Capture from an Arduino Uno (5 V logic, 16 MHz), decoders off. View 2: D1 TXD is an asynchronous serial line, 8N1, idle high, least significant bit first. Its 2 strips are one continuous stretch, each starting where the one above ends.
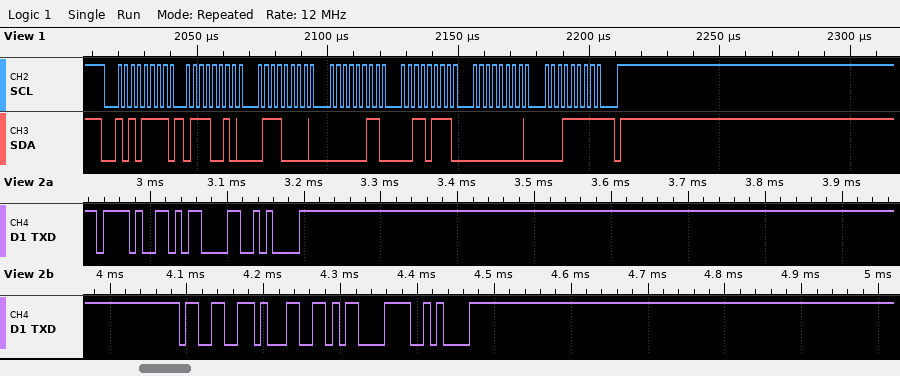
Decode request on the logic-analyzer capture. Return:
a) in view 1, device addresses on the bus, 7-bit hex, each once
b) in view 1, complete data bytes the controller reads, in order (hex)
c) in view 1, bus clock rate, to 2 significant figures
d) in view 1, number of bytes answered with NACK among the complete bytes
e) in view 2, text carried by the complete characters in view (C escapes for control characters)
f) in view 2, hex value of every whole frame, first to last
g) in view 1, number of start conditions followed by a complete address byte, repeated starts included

0x57
72 70 03 37 00 1F
400 kHz
1
"/\r\n31\r\n"
0x2F 0x0D 0x0A 0x33 0x31 0x0D 0x0A
1
